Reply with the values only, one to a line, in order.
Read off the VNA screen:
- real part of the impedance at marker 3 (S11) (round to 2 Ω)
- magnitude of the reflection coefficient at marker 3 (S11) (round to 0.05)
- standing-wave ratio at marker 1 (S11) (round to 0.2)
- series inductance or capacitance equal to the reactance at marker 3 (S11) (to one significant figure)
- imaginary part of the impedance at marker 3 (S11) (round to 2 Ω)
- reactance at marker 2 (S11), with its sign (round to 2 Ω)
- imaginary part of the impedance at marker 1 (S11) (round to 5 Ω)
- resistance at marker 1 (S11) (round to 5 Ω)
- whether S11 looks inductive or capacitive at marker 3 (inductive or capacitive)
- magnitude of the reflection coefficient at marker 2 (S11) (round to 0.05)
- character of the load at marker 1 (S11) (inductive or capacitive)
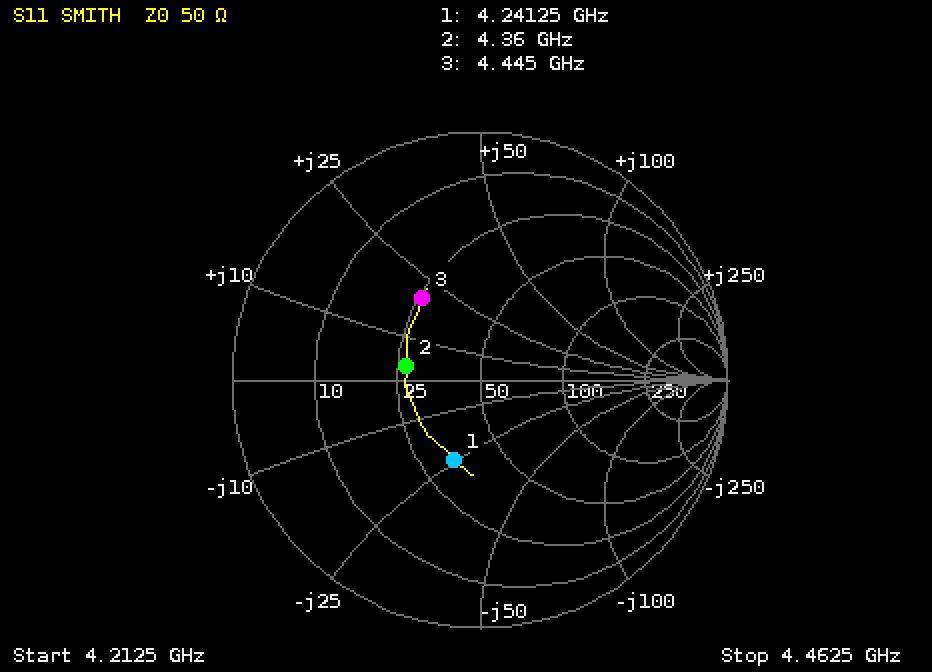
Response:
26 Ω
0.40
2.0
700 pH
+20 Ω
+4 Ω
-25 Ω
35 Ω
inductive
0.30
capacitive
